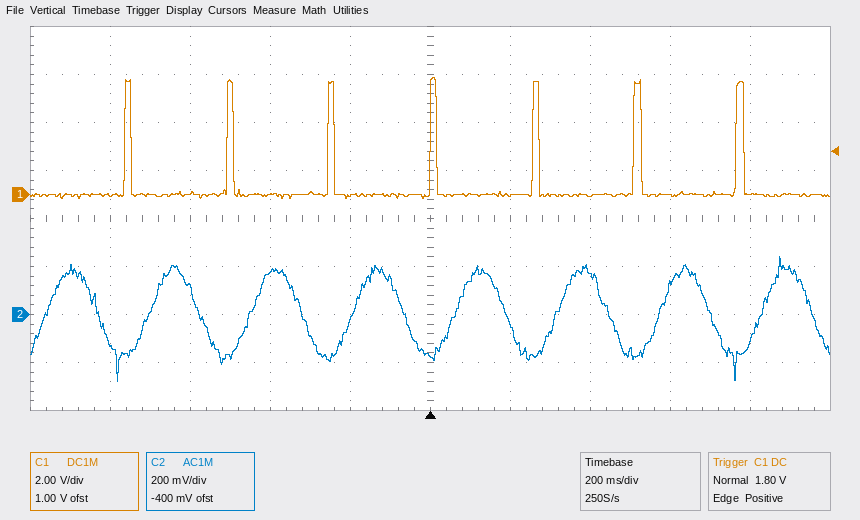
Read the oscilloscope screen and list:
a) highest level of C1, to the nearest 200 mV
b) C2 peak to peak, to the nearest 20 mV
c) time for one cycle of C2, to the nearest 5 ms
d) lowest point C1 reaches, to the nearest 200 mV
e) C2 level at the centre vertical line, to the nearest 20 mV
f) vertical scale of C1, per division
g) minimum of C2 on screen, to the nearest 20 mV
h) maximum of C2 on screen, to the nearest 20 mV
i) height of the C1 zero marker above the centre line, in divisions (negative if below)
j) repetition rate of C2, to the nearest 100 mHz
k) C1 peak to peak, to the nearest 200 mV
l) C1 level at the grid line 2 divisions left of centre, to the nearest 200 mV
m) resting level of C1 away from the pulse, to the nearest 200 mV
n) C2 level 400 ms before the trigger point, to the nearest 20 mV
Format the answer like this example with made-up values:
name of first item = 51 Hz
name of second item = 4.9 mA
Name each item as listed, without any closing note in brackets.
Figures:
highest level of C1, to the nearest 200 mV = 4.8 V
C2 peak to peak, to the nearest 20 mV = 520 mV
time for one cycle of C2, to the nearest 5 ms = 255 ms
lowest point C1 reaches, to the nearest 200 mV = -200 mV
C2 level at the centre vertical line, to the nearest 20 mV = -180 mV
vertical scale of C1, per division = 2 V
minimum of C2 on screen, to the nearest 20 mV = -280 mV
maximum of C2 on screen, to the nearest 20 mV = 240 mV
height of the C1 zero marker above the centre line, in divisions = +0.5 div
repetition rate of C2, to the nearest 100 mHz = 3.9 Hz
C1 peak to peak, to the nearest 200 mV = 5.0 V
C1 level at the grid line 2 divisions left of centre, to the nearest 200 mV = 0.0 V
resting level of C1 away from the pulse, to the nearest 200 mV = 0.0 V
C2 level 400 ms before the trigger point, to the nearest 20 mV = 180 mV
